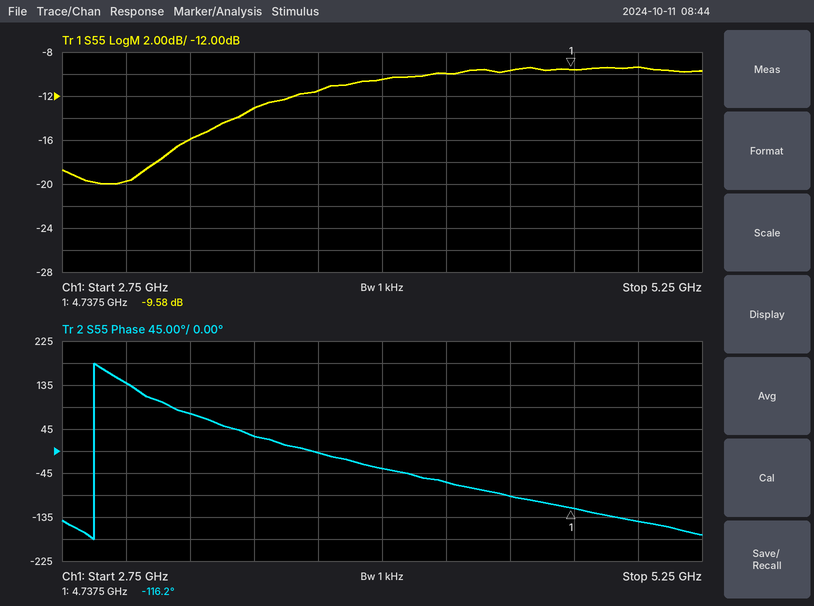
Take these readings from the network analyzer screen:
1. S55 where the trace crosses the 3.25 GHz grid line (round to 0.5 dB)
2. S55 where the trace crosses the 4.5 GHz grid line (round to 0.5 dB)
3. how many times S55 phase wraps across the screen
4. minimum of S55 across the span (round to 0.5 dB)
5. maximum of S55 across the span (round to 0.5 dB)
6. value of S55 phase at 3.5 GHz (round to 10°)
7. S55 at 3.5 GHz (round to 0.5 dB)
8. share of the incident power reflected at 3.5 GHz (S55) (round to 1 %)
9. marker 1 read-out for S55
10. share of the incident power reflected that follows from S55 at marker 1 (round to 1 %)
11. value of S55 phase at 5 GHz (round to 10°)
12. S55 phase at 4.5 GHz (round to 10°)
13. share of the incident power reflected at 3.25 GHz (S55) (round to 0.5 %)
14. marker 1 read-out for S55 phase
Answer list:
-16.0 dB
-9.5 dB
1
-20.0 dB
-9.5 dB
30°
-13.0 dB
5 %
-9.58 dB
11 %
-140°
-90°
2.5 %
-116.2°
